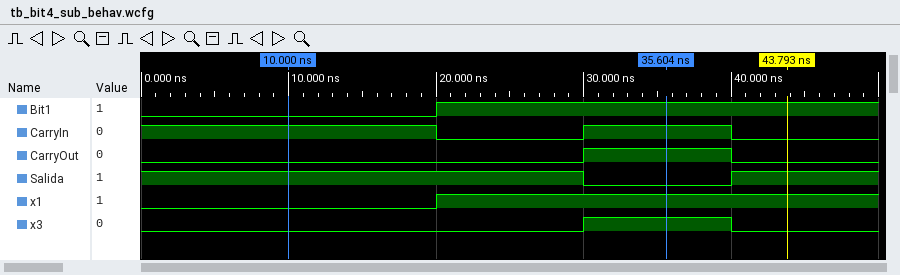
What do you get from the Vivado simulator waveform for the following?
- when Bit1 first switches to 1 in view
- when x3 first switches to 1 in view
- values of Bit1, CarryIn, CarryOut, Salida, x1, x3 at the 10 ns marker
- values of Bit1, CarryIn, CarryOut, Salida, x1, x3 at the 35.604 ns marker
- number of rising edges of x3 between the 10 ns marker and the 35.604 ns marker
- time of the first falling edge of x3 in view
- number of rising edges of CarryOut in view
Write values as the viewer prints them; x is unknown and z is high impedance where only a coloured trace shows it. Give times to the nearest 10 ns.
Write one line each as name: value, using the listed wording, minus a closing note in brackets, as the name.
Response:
when Bit1 first switches to 1 in view: 20 ns
when x3 first switches to 1 in view: 30 ns
values of Bit1, CarryIn, CarryOut, Salida, x1, x3 at the 10 ns marker: Bit1=0, CarryIn=1, CarryOut=0, Salida=1, x1=0, x3=0
values of Bit1, CarryIn, CarryOut, Salida, x1, x3 at the 35.604 ns marker: Bit1=1, CarryIn=1, CarryOut=1, Salida=0, x1=1, x3=1
number of rising edges of x3 between the 10 ns marker and the 35.604 ns marker: 1
time of the first falling edge of x3 in view: 40 ns
number of rising edges of CarryOut in view: 1
